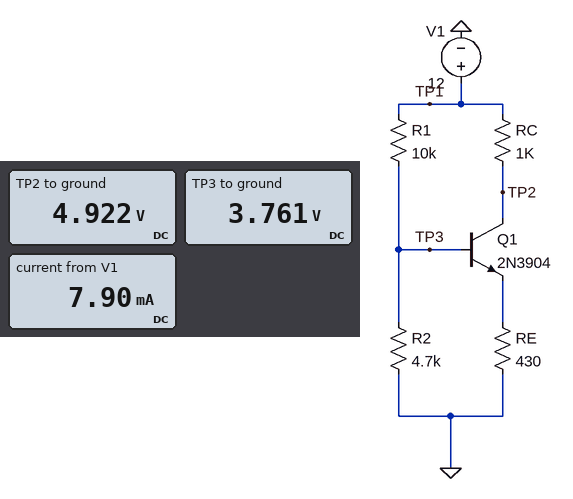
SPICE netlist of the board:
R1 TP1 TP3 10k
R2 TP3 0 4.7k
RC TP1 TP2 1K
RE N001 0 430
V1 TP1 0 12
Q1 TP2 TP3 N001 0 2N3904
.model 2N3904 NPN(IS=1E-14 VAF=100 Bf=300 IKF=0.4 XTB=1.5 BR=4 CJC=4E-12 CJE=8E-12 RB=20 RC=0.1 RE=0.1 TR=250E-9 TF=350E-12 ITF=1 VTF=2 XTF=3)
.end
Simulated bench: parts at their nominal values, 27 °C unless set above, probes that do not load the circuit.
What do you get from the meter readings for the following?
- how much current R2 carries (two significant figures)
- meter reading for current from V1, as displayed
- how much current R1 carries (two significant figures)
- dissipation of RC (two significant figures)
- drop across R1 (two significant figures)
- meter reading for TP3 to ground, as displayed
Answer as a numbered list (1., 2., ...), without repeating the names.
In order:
1. 800 µA
2. 7.90 mA
3. 820 µA
4. 50 mW
5. 8.2 V
6. 3.761 V
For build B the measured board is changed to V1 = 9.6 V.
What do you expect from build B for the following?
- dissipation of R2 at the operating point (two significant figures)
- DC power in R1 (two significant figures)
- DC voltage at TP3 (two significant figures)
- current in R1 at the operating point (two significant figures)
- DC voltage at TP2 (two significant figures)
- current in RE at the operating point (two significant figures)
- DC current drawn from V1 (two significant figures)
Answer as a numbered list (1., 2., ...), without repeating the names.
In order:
1. 1.9 mW
2. 4.3 mW
3. 3.0 V
4. 660 µA
5. 4.2 V
6. 5.4 mA
7. 6.0 mA
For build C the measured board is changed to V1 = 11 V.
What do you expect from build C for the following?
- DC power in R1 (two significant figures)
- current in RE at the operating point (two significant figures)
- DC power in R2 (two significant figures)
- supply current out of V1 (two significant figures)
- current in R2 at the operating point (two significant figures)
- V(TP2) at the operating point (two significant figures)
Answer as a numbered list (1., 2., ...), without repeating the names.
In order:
1. 5.7 mW
2. 6.4 mA
3. 2.5 mW
4. 7.1 mA
5. 730 µA
6. 4.6 V
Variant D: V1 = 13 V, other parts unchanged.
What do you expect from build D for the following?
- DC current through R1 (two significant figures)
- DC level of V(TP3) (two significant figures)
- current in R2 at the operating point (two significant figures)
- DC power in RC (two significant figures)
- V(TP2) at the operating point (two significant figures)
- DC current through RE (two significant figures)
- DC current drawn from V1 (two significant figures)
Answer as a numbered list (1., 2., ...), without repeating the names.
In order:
1. 890 µA
2. 4.1 V
3. 870 µA
4. 61 mW
5. 5.2 V
6. 7.8 mA
7. 8.7 mA
